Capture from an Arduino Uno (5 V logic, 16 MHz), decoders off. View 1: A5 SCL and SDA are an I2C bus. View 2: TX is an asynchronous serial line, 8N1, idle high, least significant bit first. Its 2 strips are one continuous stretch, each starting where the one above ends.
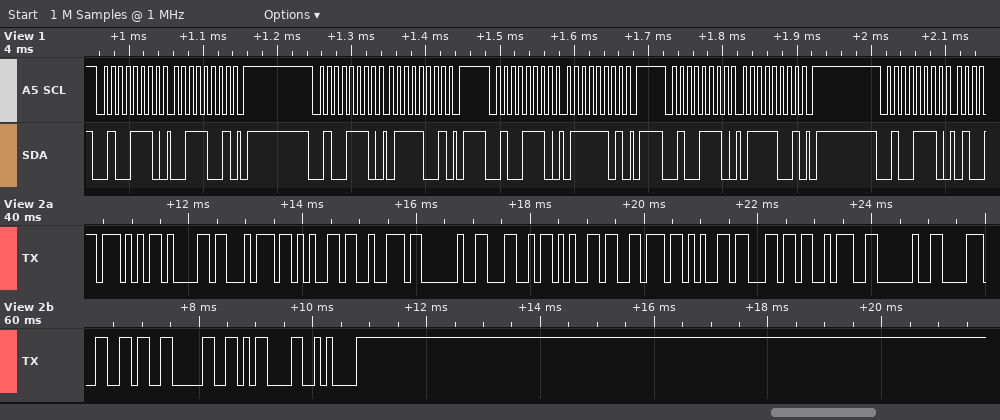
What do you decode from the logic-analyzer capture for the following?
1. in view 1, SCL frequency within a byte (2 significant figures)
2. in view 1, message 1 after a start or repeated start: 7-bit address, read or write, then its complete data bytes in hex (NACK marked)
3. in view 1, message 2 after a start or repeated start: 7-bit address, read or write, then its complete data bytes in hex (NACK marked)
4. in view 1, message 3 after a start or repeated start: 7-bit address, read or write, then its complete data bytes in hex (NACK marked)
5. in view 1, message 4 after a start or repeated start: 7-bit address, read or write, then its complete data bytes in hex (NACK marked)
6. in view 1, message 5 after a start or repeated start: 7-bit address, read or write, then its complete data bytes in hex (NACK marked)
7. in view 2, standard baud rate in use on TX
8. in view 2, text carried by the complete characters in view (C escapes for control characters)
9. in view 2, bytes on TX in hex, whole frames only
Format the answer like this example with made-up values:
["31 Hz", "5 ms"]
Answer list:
["100 kHz", "0x27 write: 39", "0x27 write: 79", "0x27 write: 7D", "0x27 write: 79", "0x27 write", "9600 baud", "\"Water Level: 860\\r\\n\"", "57 61 74 65 72 20 4C 65 76 65 6C 3A 20 38 36 30 0D 0A"]
